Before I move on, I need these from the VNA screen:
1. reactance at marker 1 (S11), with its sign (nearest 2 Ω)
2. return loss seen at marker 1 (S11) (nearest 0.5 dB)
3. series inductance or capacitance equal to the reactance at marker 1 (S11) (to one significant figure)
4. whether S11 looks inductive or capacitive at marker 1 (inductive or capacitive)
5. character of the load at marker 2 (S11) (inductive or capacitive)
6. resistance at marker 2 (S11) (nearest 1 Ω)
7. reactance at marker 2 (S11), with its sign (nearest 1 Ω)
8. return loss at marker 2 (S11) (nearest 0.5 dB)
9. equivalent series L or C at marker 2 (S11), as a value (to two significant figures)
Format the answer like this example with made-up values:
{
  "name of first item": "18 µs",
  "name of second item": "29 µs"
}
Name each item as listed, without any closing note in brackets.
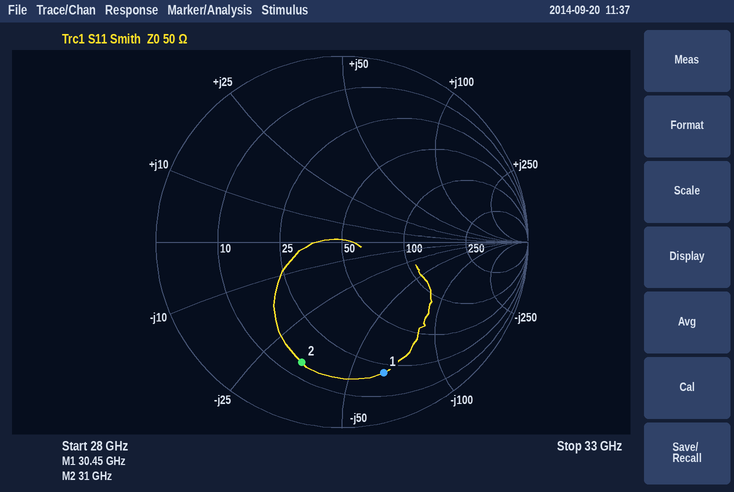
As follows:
{
  "reactance at marker 1 (S11), with its sign": "-64 Ω",
  "return loss seen at marker 1 (S11)": "2.5 dB",
  "series inductance or capacitance equal to the reactance at marker 1 (S11)": "80 fF",
  "whether S11 looks inductive or capacitive at marker 1": "capacitive",
  "character of the load at marker 2 (S11)": "capacitive",
  "resistance at marker 2 (S11)": "14 Ω",
  "reactance at marker 2 (S11), with its sign": "-34 Ω",
  "return loss at marker 2 (S11)": "3.5 dB",
  "equivalent series L or C at marker 2 (S11), as a value": "150 fF"
}
